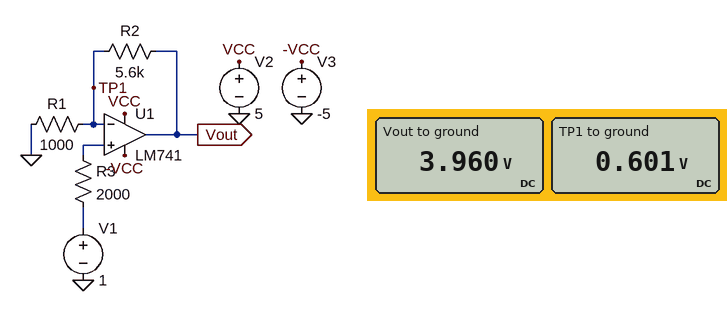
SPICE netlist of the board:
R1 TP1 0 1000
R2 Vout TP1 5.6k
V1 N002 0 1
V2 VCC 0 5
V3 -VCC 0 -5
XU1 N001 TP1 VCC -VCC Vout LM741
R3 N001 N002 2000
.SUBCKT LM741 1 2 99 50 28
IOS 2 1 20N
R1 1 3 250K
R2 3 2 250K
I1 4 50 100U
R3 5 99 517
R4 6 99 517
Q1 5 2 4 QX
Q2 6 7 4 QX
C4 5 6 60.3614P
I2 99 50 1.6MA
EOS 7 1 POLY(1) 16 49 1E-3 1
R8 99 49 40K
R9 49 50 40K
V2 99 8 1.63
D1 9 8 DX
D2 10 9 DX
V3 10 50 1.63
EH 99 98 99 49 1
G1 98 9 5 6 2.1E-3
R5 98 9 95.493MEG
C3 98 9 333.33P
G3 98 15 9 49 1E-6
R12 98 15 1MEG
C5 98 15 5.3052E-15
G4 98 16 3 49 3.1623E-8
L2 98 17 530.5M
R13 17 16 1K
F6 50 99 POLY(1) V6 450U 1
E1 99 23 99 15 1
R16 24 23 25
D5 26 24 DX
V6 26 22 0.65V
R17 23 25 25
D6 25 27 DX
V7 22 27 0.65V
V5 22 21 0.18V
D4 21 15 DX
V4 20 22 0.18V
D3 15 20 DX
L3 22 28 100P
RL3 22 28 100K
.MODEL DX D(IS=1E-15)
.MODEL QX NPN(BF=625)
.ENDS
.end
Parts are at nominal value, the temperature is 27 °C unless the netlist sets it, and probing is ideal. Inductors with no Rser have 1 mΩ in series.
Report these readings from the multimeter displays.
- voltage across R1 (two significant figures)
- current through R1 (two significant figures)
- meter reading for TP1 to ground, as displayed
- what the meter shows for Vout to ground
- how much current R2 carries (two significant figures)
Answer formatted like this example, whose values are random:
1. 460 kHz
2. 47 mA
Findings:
1. 600 mV
2. 600 µA
3. 0.601 V
4. 3.960 V
5. 600 µA
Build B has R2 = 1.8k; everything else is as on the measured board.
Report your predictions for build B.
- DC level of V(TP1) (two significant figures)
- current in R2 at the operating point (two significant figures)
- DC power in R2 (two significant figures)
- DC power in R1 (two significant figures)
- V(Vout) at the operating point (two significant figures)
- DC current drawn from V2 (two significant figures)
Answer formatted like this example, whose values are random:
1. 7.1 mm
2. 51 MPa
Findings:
1. 1.0 V
2. 1.0 mA
3. 1.8 mW
4. 1.0 mW
5. 2.8 V
6. 2.4 mA
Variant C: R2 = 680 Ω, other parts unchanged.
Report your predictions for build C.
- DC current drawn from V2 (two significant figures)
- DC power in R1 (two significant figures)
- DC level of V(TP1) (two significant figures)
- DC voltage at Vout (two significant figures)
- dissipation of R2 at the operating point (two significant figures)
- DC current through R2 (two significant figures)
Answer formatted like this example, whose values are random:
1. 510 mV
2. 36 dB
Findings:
1. 2.4 mA
2. 1.0 mW
3. 1.0 V
4. 1.7 V
5. 680 µW
6. 1.0 mA
